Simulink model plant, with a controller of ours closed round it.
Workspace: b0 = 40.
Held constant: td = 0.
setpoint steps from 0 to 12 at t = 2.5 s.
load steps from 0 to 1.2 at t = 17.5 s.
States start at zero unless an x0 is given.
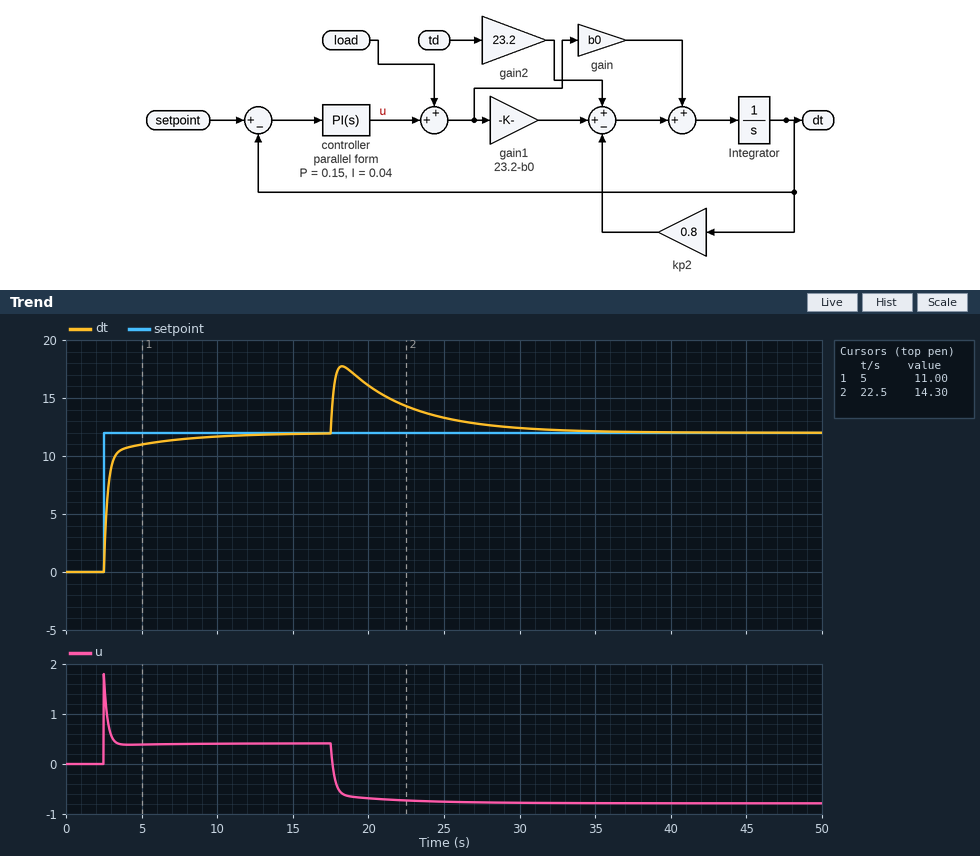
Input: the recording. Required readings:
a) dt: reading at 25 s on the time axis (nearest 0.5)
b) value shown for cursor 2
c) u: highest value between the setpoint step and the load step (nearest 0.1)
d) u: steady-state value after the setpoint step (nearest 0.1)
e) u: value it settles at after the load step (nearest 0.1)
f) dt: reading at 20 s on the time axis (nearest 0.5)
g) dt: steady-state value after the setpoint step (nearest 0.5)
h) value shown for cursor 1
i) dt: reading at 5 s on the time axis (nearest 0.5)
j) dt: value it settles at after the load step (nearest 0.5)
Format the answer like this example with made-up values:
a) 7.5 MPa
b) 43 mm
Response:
a) 13.5
b) 14.30
c) 1.8
d) 0.4
e) -0.8
f) 16.0
g) 12.0
h) 11.00
i) 11.0
j) 12.0
